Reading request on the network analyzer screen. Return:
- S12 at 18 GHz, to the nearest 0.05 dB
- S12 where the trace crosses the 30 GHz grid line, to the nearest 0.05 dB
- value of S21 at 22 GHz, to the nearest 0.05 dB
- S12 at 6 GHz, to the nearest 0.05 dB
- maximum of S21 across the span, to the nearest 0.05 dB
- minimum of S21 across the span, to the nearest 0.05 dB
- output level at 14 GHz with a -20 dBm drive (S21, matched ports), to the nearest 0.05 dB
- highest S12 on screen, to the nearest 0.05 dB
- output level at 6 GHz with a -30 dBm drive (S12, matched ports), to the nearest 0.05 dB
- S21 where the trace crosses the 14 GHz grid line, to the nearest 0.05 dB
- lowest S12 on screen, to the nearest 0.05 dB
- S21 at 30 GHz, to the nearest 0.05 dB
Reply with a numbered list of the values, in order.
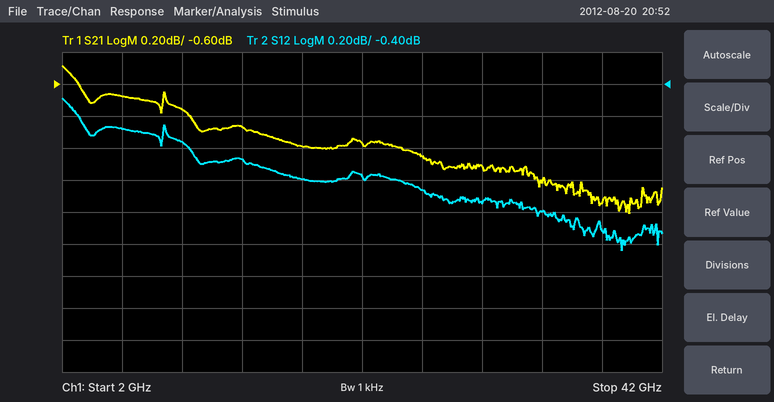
1. -1.00 dB
2. -1.15 dB
3. -0.95 dB
4. -0.70 dB
5. -0.50 dB
6. -1.40 dB
7. -20.85 dBm
8. -0.50 dB
9. -30.70 dBm
10. -0.85 dB
11. -1.45 dB
12. -1.10 dB
